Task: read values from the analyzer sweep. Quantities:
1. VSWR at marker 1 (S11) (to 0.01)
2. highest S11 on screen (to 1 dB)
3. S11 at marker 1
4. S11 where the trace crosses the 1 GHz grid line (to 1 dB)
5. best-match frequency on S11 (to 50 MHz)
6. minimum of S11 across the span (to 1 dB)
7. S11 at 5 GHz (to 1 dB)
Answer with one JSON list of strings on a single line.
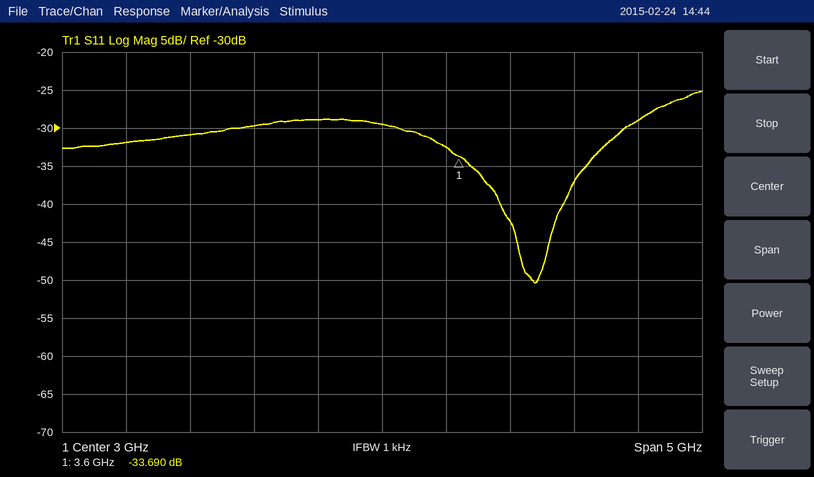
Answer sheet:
["1.04", "-25 dB", "-33.690 dB", "-32 dB", "4.20 GHz", "-50 dB", "-29 dB"]
